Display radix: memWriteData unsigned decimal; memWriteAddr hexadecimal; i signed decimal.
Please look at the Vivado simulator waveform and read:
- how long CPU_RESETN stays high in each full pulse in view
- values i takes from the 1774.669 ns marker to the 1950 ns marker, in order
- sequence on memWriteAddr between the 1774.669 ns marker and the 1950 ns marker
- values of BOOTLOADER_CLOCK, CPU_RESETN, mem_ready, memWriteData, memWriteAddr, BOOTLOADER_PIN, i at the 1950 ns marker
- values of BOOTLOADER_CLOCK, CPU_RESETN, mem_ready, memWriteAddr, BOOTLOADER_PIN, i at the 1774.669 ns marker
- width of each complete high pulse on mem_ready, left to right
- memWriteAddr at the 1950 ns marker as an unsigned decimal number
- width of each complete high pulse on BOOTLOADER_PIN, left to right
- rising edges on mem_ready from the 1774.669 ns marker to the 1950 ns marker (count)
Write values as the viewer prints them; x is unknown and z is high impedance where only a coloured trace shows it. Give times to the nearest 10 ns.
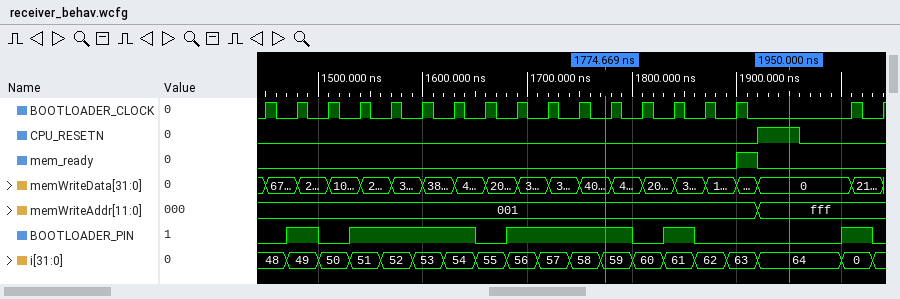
40 ns
59, 60, 61, 62, 63, 64
001, fff
BOOTLOADER_CLOCK=0, CPU_RESETN=1, mem_ready=0, memWriteData=0, memWriteAddr=fff, BOOTLOADER_PIN=0, i=64
BOOTLOADER_CLOCK=0, CPU_RESETN=0, mem_ready=0, memWriteAddr=001, BOOTLOADER_PIN=1, i=59
20 ns
4095
30 ns, 120 ns, 120 ns, 30 ns, 30 ns
1
